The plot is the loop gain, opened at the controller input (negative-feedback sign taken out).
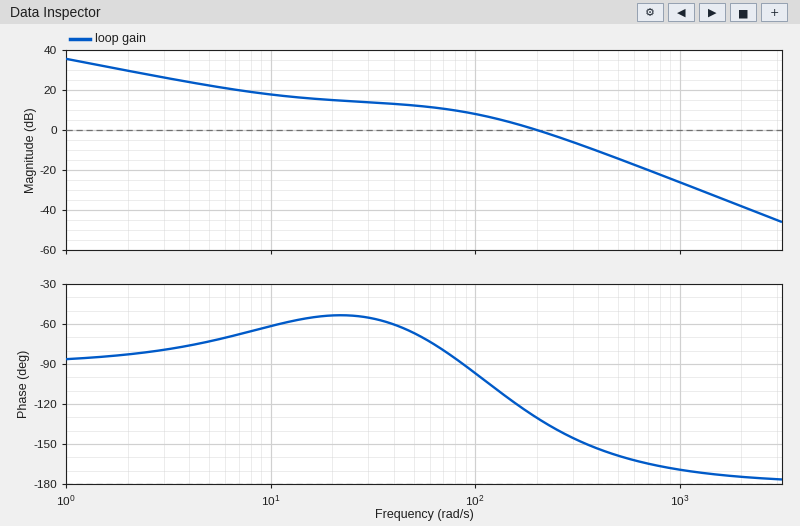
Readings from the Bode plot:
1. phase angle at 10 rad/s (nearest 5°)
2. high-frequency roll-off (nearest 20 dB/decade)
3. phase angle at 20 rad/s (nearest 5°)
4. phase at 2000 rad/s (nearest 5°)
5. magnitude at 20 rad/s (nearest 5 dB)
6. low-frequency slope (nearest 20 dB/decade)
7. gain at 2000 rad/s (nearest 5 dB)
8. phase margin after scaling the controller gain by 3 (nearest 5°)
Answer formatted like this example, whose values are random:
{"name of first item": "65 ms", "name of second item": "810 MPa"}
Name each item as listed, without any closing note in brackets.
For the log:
{"phase angle at 10 rad/s": "-60°", "high-frequency roll-off": "-40 dB/decade", "phase angle at 20 rad/s": "-55°", "phase at 2000 rad/s": "-175°", "magnitude at 20 rad/s": "15 dB", "low-frequency slope": "-20 dB/decade", "gain at 2000 rad/s": "-40 dB", "phase margin after scaling the controller gain by 3": "30°"}
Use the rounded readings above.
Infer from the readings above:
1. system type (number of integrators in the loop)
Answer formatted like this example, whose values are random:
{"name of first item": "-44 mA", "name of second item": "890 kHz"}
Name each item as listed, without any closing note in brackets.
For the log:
{"system type": "1"}
